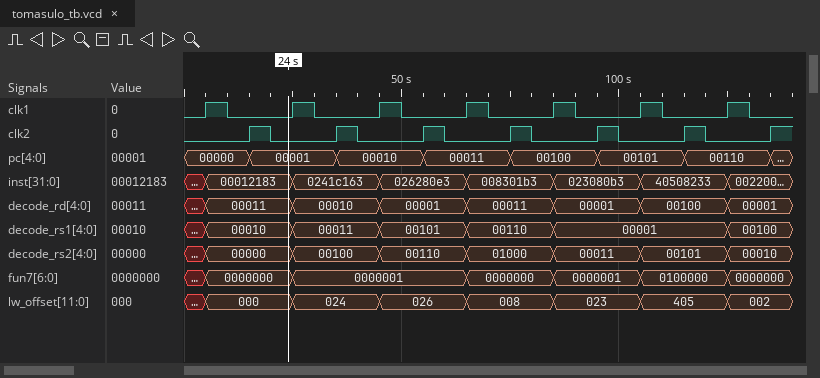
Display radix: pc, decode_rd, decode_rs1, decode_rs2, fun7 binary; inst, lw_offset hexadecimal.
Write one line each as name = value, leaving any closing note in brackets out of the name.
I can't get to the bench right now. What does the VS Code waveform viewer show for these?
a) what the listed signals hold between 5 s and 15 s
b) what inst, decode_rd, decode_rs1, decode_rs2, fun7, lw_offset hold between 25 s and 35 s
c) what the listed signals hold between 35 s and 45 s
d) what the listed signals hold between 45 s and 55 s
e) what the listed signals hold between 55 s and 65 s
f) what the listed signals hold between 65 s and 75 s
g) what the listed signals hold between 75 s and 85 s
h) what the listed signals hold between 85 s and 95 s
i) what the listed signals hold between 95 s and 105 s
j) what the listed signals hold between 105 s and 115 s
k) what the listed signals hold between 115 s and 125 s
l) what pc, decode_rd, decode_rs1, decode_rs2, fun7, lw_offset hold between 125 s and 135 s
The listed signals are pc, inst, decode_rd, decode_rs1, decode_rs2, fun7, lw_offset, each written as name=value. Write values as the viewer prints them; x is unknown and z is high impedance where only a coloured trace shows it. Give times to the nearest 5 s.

what the listed signals hold between 5 s and 15 s = pc=00000, inst=00012183, decode_rd=00011, decode_rs1=00010, decode_rs2=00000, fun7=0000000, lw_offset=000
what inst, decode_rd, decode_rs1, decode_rs2, fun7, lw_offset hold between 25 s and 35 s = inst=0241c163, decode_rd=00010, decode_rs1=00011, decode_rs2=00100, fun7=0000001, lw_offset=024
what the listed signals hold between 35 s and 45 s = pc=00010, inst=0241c163, decode_rd=00010, decode_rs1=00011, decode_rs2=00100, fun7=0000001, lw_offset=024
what the listed signals hold between 45 s and 55 s = pc=00010, inst=026280e3, decode_rd=00001, decode_rs1=00101, decode_rs2=00110, fun7=0000001, lw_offset=026
what the listed signals hold between 55 s and 65 s = pc=00011, inst=026280e3, decode_rd=00001, decode_rs1=00101, decode_rs2=00110, fun7=0000001, lw_offset=026
what the listed signals hold between 65 s and 75 s = pc=00011, inst=008301b3, decode_rd=00011, decode_rs1=00110, decode_rs2=01000, fun7=0000000, lw_offset=008
what the listed signals hold between 75 s and 85 s = pc=00100, inst=008301b3, decode_rd=00011, decode_rs1=00110, decode_rs2=01000, fun7=0000000, lw_offset=008
what the listed signals hold between 85 s and 95 s = pc=00100, inst=023080b3, decode_rd=00001, decode_rs1=00001, decode_rs2=00011, fun7=0000001, lw_offset=023
what the listed signals hold between 95 s and 105 s = pc=00101, inst=023080b3, decode_rd=00001, decode_rs1=00001, decode_rs2=00011, fun7=0000001, lw_offset=023
what the listed signals hold between 105 s and 115 s = pc=00101, inst=40508233, decode_rd=00100, decode_rs1=00001, decode_rs2=00101, fun7=0100000, lw_offset=405
what the listed signals hold between 115 s and 125 s = pc=00110, inst=40508233, decode_rd=00100, decode_rs1=00001, decode_rs2=00101, fun7=0100000, lw_offset=405
what pc, decode_rd, decode_rs1, decode_rs2, fun7, lw_offset hold between 125 s and 135 s = pc=00110, decode_rd=00001, decode_rs1=00100, decode_rs2=00010, fun7=0000000, lw_offset=002
